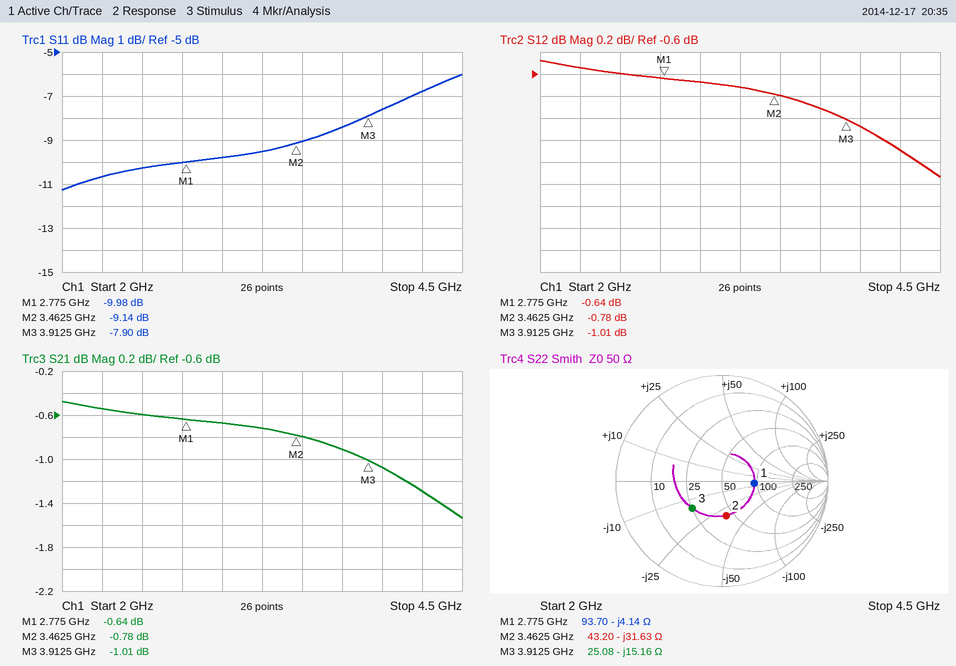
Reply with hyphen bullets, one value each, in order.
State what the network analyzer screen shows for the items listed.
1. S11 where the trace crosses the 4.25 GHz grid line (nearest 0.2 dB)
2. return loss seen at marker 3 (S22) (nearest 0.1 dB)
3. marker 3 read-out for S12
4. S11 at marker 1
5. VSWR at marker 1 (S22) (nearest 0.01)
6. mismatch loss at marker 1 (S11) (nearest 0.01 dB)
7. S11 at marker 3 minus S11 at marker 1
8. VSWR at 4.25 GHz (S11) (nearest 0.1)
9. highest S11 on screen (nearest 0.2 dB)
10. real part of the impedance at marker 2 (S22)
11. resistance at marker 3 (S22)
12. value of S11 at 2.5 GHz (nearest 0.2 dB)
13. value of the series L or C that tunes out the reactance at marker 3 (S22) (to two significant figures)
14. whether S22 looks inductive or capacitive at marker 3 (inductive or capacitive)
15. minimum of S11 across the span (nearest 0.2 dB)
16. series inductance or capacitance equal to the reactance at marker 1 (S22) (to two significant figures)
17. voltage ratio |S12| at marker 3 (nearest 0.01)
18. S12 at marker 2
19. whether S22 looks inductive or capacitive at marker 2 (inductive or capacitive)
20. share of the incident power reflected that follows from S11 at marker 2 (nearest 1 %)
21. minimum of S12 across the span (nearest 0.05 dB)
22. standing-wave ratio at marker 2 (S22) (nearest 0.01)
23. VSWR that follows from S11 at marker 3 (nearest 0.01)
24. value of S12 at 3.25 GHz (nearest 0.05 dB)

- -6.8 dB
- 8.4 dB
- -1.01 dB
- -9.98 dB
- 1.88
- 0.46 dB
- 2.08 dB
- 2.7
- -6.0 dB
- 43.20 Ω
- 25.08 Ω
- -10.2 dB
- 620 pH
- capacitive
- -11.2 dB
- 14 pF
- 0.89
- -0.78 dB
- capacitive
- 12 %
- -1.55 dB
- 1.98
- 2.35
- -0.70 dB
